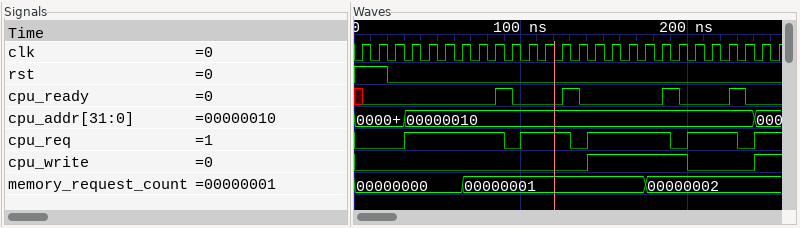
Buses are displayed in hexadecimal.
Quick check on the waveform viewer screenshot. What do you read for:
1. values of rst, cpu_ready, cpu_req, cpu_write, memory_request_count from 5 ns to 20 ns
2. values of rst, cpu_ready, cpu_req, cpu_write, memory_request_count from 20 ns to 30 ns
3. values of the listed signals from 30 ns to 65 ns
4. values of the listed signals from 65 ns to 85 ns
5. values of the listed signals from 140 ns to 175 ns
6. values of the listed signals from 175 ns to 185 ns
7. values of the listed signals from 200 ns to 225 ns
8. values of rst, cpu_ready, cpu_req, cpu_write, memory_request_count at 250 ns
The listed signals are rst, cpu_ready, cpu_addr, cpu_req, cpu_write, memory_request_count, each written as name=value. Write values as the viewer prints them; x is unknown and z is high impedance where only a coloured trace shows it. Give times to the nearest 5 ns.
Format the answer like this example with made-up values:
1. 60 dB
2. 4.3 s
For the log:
1. rst=1, cpu_ready=0, cpu_req=0, cpu_write=0, memory_request_count=00000000
2. rst=0, cpu_ready=0, cpu_req=0, cpu_write=0, memory_request_count=00000000
3. rst=0, cpu_ready=0, cpu_addr=00000010, cpu_req=1, cpu_write=0, memory_request_count=00000000
4. rst=0, cpu_ready=0, cpu_addr=00000010, cpu_req=1, cpu_write=0, memory_request_count=00000001
5. rst=0, cpu_ready=0, cpu_addr=00000010, cpu_req=1, cpu_write=1, memory_request_count=00000001
6. rst=0, cpu_ready=0, cpu_addr=00000010, cpu_req=1, cpu_write=1, memory_request_count=00000002
7. rst=0, cpu_ready=0, cpu_addr=00000010, cpu_req=1, cpu_write=0, memory_request_count=00000002
8. rst=0, cpu_ready=0, cpu_req=1, cpu_write=1, memory_request_count=00000002
